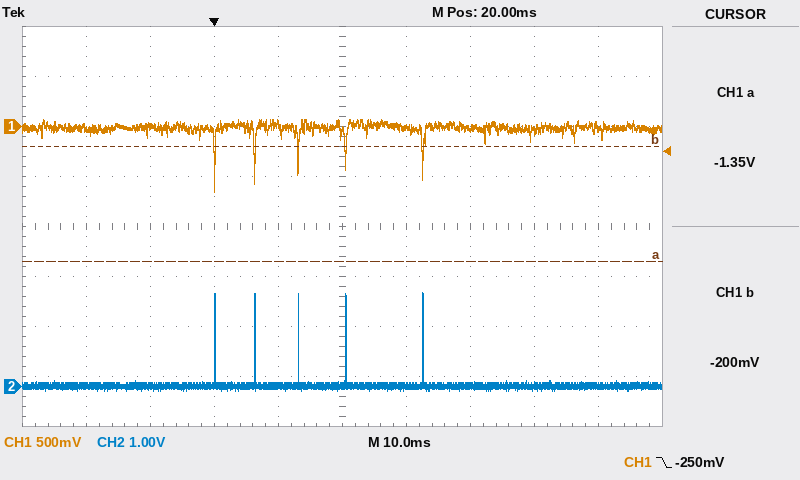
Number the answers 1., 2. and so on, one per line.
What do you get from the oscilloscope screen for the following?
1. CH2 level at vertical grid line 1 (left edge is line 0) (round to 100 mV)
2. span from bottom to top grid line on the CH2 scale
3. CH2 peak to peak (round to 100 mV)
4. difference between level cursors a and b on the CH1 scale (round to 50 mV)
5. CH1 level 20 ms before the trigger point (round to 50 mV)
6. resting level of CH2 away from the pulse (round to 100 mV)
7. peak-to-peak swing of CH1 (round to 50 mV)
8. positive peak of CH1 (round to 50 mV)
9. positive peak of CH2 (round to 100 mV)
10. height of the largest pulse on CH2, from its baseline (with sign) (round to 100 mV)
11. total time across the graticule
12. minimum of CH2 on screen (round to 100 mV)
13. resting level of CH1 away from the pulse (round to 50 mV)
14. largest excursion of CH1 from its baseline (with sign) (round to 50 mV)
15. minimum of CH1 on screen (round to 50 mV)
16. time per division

1. 0.0 V
2. 8 V
3. 2.0 V
4. 1.15 V
5. 0 mV
6. 0.0 V
7. 700 mV
8. 50 mV
9. 1.9 V
10. +1.9 V
11. 100 ms
12. -100 mV
13. 0 mV
14. -650 mV
15. -650 mV
16. 10 ms
